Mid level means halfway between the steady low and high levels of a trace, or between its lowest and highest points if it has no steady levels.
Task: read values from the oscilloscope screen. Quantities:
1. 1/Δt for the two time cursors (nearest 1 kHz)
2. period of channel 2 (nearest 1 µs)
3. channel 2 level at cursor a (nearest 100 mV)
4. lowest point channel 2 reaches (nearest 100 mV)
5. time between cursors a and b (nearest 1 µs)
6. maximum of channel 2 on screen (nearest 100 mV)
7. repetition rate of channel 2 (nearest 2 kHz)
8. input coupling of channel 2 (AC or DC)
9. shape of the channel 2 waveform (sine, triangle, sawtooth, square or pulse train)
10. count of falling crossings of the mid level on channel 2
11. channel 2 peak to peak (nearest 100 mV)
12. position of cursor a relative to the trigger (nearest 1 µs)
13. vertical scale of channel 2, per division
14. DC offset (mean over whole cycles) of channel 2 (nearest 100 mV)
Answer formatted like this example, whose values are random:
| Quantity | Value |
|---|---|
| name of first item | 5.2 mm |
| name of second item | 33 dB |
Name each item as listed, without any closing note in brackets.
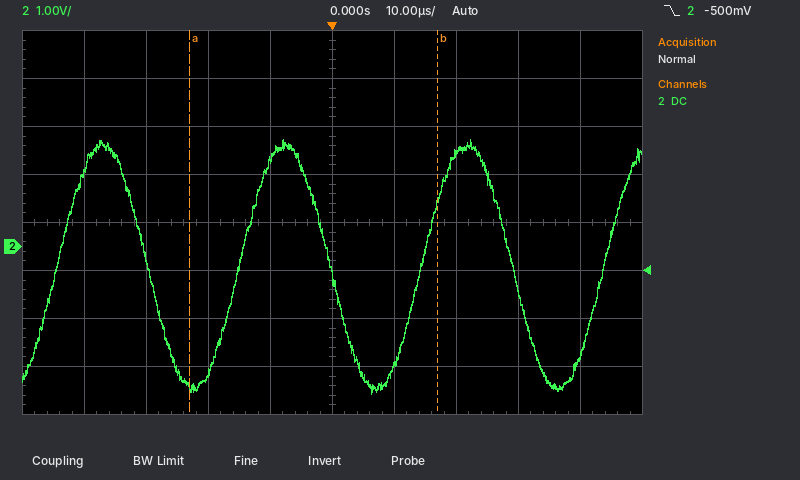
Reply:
| Quantity | Value |
|---|---|
| 1/Δt for the two time cursors | 25 kHz |
| period of channel 2 | 29 µs |
| channel 2 level at cursor a | -2.9 V |
| lowest point channel 2 reaches | -3.1 V |
| time between cursors a and b | 40 µs |
| maximum of channel 2 on screen | 2.2 V |
| repetition rate of channel 2 | 34 kHz |
| input coupling of channel 2 | DC |
| shape of the channel 2 waveform | sine |
| count of falling crossings of the mid level on channel 2 | 3 |
| channel 2 peak to peak | 5.3 V |
| position of cursor a relative to the trigger | -23 µs |
| vertical scale of channel 2, per division | 1 V |
| DC offset (mean over whole cycles) of channel 2 | -400 mV |
